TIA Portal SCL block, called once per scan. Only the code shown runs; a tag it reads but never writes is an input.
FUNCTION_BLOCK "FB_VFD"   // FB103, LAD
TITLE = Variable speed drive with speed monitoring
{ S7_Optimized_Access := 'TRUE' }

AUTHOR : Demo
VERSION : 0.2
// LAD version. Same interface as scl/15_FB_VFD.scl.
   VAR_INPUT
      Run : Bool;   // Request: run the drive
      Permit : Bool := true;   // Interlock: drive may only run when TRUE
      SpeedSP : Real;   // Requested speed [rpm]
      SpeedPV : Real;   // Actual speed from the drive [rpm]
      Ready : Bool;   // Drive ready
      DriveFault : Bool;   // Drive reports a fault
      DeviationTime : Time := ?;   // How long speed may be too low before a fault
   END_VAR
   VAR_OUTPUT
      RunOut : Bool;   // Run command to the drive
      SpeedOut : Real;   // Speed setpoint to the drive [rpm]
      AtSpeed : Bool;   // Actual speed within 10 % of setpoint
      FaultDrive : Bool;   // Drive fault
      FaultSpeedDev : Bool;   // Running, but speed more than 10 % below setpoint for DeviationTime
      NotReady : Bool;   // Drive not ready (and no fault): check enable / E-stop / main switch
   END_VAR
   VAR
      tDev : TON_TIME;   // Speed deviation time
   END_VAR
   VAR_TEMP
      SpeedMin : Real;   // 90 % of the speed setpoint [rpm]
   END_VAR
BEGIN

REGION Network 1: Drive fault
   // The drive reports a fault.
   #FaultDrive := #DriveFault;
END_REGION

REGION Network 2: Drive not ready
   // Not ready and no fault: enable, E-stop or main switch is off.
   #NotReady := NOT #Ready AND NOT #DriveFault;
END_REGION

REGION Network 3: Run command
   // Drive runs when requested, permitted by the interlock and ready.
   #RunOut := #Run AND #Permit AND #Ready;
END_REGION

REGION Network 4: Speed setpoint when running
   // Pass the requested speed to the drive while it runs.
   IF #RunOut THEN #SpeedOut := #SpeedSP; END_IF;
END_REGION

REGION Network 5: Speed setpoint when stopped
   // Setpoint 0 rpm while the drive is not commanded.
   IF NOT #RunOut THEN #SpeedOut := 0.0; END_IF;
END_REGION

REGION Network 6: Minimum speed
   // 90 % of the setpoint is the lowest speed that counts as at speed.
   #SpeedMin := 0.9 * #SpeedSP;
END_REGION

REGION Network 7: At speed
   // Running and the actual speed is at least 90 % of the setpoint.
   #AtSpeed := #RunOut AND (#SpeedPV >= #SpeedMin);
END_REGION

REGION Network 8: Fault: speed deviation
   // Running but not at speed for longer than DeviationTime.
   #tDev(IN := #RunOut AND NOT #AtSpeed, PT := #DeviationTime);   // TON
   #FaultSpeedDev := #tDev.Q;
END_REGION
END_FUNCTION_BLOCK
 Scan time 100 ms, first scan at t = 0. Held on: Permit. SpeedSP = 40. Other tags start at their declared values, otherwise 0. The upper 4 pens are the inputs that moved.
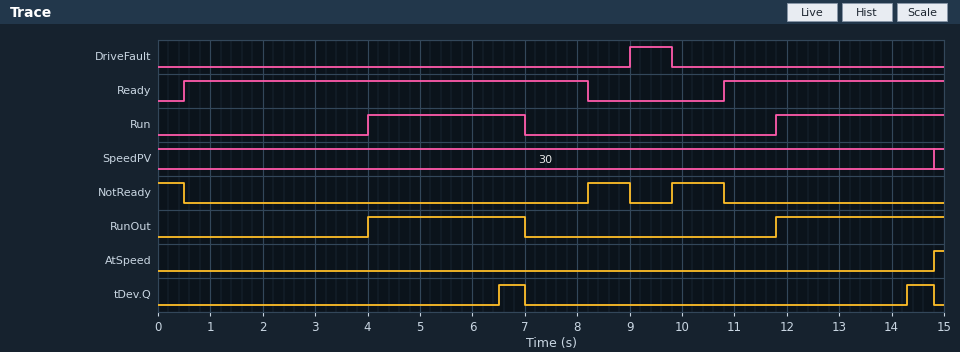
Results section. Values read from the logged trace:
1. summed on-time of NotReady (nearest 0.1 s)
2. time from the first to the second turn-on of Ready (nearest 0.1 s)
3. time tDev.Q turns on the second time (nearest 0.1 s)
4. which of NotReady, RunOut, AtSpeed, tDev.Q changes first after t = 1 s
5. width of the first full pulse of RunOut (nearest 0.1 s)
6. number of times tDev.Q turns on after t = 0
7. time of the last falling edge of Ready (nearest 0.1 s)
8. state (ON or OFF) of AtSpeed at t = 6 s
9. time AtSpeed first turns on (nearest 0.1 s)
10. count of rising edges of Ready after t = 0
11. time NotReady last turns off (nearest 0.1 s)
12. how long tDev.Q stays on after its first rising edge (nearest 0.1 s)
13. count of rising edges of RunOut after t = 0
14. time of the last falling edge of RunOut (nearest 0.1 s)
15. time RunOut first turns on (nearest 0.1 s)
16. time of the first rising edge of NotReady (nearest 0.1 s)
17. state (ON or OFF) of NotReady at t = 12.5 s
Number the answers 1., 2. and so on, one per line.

1. 2.3 s
2. 10.3 s
3. 14.3 s
4. RunOut
5. 3.0 s
6. 2
7. 8.2 s
8. OFF
9. 14.8 s
10. 2
11. 10.8 s
12. 0.5 s
13. 2
14. 7.0 s
15. 4.0 s
16. 8.2 s
17. OFF
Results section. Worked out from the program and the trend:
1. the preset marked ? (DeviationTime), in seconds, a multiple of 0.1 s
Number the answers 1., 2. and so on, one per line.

1. 2.5 s
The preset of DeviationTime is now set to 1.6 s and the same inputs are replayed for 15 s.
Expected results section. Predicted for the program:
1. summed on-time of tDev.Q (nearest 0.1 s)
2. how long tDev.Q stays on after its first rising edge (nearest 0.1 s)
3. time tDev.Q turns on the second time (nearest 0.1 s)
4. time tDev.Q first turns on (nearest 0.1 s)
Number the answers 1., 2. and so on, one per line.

1. 2.8 s
2. 1.4 s
3. 13.4 s
4. 5.6 s
